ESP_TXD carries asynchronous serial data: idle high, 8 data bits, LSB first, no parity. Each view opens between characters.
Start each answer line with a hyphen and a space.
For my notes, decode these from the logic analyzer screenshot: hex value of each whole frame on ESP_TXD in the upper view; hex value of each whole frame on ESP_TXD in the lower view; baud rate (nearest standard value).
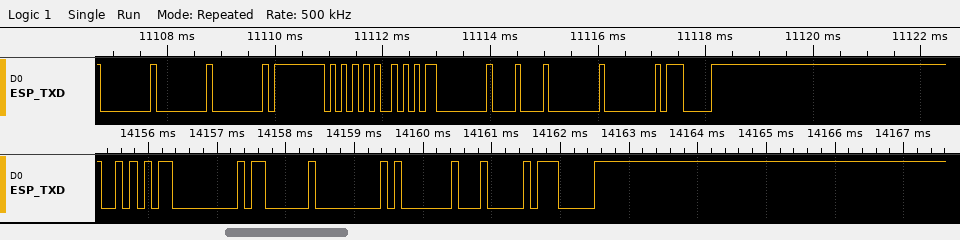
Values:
- 00, 00, 00, FF, 55, AA, 00, 08, 00, 00, 07
- AA, 00, 03, 00, 01, 04, 07
- 9600 baud
